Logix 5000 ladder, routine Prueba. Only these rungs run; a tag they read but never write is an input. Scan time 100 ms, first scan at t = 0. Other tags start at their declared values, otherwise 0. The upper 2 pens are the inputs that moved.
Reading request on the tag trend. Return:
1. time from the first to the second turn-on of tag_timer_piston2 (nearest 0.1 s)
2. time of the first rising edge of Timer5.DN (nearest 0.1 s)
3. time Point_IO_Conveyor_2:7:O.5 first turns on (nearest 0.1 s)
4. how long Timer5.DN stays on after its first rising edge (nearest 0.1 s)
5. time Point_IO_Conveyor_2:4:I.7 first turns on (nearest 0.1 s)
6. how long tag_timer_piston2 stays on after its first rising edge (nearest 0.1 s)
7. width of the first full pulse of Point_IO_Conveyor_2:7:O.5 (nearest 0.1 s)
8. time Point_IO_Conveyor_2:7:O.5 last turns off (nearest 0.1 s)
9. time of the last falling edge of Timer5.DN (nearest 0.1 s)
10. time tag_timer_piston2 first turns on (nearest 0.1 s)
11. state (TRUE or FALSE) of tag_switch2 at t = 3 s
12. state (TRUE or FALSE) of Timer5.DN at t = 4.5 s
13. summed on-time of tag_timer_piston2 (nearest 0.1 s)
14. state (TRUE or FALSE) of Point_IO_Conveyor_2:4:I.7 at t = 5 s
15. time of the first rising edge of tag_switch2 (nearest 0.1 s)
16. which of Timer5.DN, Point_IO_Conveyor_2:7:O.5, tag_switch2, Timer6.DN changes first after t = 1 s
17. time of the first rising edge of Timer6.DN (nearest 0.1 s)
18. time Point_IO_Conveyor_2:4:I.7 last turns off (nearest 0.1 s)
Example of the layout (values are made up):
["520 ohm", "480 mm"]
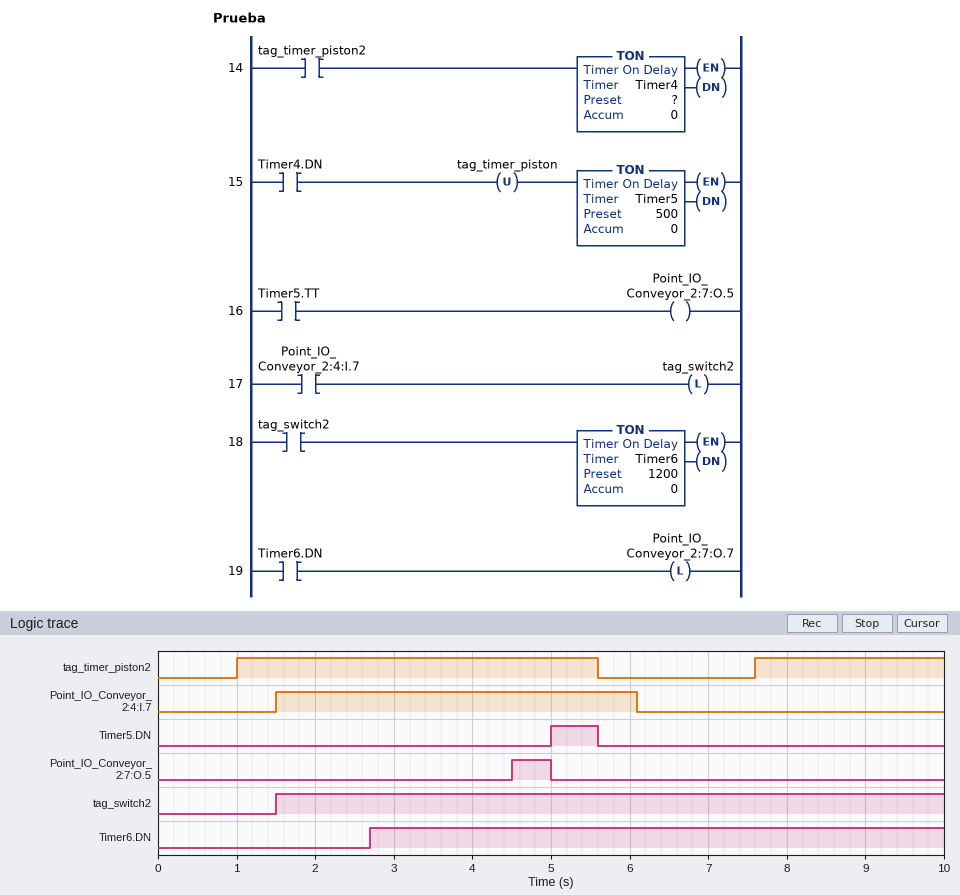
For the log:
["6.6 s", "5.0 s", "4.5 s", "0.6 s", "1.5 s", "4.6 s", "0.5 s", "5.0 s", "5.6 s", "1.0 s", "TRUE", "FALSE", "7.0 s", "TRUE", "1.5 s", "tag_switch2", "2.7 s", "6.1 s"]
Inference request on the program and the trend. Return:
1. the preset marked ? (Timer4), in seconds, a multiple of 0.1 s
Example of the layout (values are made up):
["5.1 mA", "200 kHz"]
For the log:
["3.5 s"]
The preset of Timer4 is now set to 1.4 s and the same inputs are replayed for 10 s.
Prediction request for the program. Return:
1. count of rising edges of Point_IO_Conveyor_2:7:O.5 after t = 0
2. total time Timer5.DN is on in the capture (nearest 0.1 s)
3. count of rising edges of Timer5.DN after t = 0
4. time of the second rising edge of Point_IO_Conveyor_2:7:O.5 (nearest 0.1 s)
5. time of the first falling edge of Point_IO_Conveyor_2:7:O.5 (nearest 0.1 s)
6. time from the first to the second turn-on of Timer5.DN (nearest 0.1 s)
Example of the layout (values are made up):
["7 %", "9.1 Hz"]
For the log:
["2", "3.2 s", "2", "9.0 s", "2.9 s", "6.6 s"]
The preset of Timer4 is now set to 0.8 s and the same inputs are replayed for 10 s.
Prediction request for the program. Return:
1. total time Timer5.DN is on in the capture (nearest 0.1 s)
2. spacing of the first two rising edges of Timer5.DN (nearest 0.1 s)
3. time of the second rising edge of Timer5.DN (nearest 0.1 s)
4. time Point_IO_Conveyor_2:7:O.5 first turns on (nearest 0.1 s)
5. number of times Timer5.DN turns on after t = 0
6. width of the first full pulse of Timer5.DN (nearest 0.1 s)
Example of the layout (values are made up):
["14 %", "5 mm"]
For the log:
["4.4 s", "6.6 s", "8.9 s", "1.8 s", "2", "3.3 s"]
